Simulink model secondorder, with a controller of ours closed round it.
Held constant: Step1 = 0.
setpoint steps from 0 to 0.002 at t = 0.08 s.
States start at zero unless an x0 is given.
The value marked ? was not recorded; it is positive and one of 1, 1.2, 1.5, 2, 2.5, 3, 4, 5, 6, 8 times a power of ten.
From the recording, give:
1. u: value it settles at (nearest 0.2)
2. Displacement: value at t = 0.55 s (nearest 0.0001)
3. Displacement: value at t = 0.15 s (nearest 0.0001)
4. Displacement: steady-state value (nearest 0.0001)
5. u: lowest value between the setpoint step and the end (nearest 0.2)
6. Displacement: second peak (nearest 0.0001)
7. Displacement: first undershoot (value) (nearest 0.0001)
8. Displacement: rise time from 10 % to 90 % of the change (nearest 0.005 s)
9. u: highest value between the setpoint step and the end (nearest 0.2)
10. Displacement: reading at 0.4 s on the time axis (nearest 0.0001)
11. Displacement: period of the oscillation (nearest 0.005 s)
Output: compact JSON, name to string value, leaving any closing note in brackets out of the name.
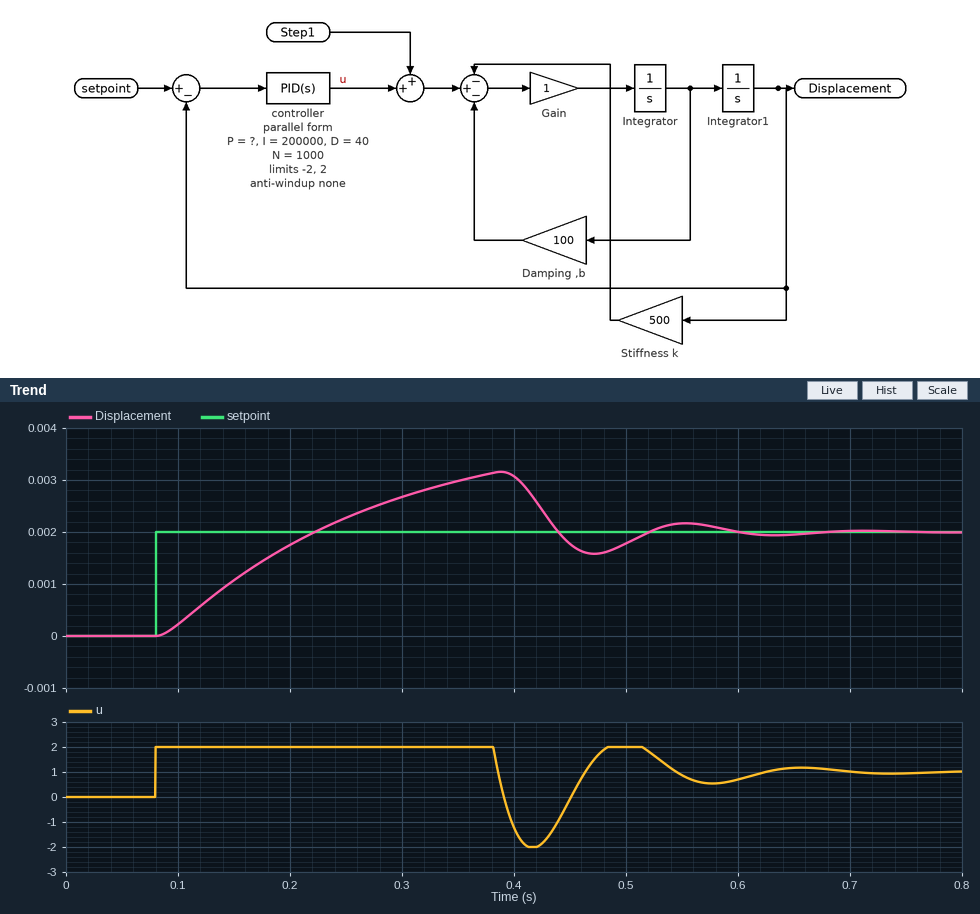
{"u: value it settles at": "1.0", "Displacement: value at t = 0.55 s": "0.0022", "Displacement: value at t = 0.15 s": "0.0011", "Displacement: steady-state value": "0.0020", "u: lowest value between the setpoint step and the end": "-2.0", "Displacement: second peak": "0.0022", "Displacement: first undershoot (value)": "0.0016", "Displacement: rise time from 10 % to 90 % of the change": "0.105 s", "u: highest value between the setpoint step and the end": "2.0", "Displacement: reading at 0.4 s on the time axis": "0.0031", "Displacement: period of the oscillation": "0.165 s"}
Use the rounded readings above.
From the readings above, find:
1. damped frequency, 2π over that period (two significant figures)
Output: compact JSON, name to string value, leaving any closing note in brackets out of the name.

{"damped frequency, 2π over that period": "38 rad/s"}
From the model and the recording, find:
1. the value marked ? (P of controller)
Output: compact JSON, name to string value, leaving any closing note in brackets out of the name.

{"the value marked ?": "4000"}
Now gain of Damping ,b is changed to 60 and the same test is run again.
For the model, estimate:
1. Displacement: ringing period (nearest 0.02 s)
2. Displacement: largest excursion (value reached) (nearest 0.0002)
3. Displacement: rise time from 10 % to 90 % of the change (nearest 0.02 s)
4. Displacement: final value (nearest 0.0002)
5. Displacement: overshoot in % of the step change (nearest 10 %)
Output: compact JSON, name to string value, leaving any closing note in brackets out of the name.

{"Displacement: ringing period": "0.14 s", "Displacement: largest excursion (value reached)": "0.0032", "Displacement: rise time from 10 % to 90 % of the change": "0.06 s", "Displacement: final value": "0.0020", "Displacement: overshoot in % of the step change": "60 %"}
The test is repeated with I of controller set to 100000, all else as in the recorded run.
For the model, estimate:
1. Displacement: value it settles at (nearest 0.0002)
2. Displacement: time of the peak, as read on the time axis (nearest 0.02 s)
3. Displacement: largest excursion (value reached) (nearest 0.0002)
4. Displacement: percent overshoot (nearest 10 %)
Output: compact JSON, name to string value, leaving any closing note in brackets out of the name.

{"Displacement: value it settles at": "0.0020", "Displacement: time of the peak, as read on the time axis": "0.36 s", "Displacement: largest excursion (value reached)": "0.0030", "Displacement: percent overshoot": "50 %"}
